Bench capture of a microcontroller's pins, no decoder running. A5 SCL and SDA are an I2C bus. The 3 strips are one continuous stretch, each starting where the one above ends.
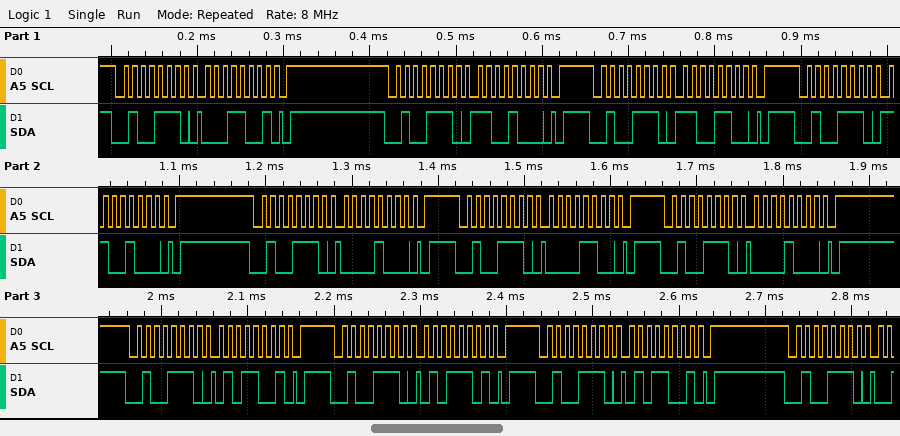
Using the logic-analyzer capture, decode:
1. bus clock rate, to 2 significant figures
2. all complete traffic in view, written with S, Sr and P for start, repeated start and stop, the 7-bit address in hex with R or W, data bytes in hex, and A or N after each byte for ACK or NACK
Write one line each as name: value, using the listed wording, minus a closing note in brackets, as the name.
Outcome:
bus clock rate, to 2 significant figures: 100 kHz
all complete traffic in view, written with S, Sr and P for start, repeated start and stop, the 7-bit address in hex with R or W, data bytes in hex, and A or N after each byte for ACK or NACK: S 27W A 19 A P S 27W A C8 A P S 27W A CC A P S 27W A C8 A P S 27W A 08 A P S 27W A 0C A P S 27W A 08 A P S 27W A 59 A P S 27W A 5D A P S 27W A 59 A P S 27W A
